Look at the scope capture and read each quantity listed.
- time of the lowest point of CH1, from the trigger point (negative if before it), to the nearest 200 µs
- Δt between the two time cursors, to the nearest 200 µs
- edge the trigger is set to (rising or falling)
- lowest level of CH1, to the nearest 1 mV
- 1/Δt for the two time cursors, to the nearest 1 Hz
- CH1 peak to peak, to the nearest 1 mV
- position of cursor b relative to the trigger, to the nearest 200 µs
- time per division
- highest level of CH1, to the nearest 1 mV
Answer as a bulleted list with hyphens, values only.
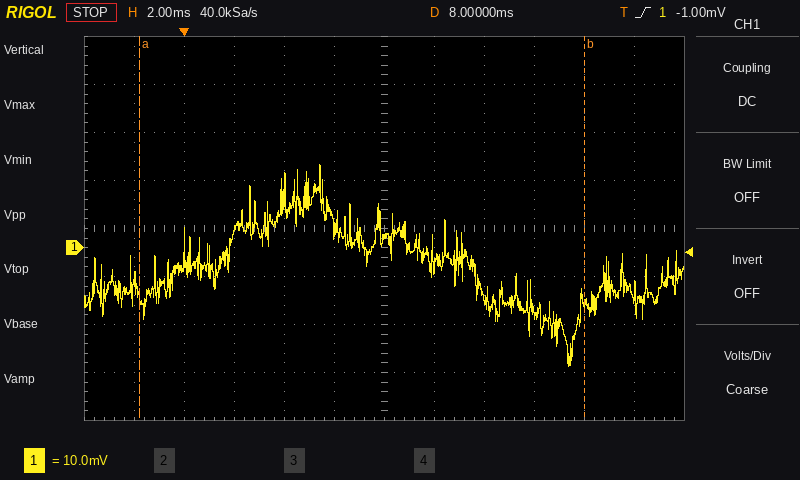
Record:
- +15.4 ms
- 17.8 ms
- rising
- -25 mV
- 56 Hz
- 42 mV
- +16.0 ms
- 2 ms
- 17 mV
